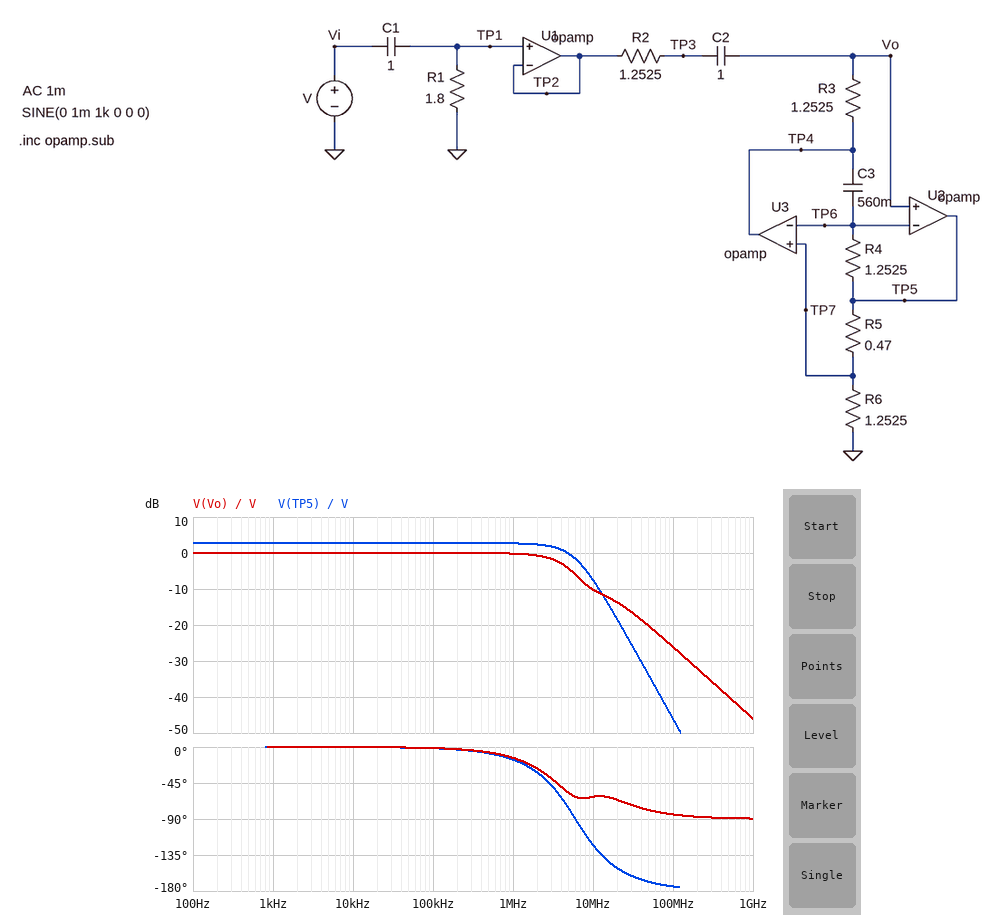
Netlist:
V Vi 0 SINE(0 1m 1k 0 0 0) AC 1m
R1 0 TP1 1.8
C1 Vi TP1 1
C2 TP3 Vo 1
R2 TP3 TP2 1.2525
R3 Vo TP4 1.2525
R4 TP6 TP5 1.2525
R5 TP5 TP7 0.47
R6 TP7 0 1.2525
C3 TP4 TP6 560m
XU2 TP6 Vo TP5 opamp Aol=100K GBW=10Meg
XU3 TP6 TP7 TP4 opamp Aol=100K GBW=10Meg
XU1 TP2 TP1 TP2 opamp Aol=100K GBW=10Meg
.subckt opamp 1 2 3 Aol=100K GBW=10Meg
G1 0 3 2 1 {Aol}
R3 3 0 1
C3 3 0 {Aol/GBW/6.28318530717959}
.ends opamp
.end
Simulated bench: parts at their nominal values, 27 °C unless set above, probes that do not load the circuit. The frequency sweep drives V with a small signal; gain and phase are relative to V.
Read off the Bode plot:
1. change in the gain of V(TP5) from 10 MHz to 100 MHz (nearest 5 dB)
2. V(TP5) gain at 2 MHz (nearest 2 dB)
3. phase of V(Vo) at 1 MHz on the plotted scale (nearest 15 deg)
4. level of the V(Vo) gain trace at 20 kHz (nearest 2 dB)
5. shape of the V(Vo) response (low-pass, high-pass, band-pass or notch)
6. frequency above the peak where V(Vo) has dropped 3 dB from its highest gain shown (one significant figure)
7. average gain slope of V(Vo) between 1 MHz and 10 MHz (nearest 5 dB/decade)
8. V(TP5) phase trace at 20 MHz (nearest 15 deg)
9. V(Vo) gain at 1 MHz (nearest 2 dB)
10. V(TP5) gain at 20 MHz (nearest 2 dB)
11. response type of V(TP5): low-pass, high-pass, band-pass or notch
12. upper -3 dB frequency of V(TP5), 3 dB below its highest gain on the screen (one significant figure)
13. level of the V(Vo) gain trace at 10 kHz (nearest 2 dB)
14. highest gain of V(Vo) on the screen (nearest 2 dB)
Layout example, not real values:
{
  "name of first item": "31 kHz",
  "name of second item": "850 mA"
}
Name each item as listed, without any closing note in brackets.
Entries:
{
  "change in the gain of V(TP5) from 10 MHz to 100 MHz": "-40 dB",
  "V(TP5) gain at 2 MHz": "2 dB",
  "phase of V(Vo) at 1 MHz on the plotted scale": "-15 deg",
  "level of the V(Vo) gain trace at 20 kHz": "0 dB",
  "shape of the V(Vo) response": "low-pass",
  "frequency above the peak where V(Vo) has dropped 3 dB from its highest gain shown": "4 MHz",
  "average gain slope of V(Vo) between 1 MHz and 10 MHz": "-10 dB/decade",
  "V(TP5) phase trace at 20 MHz": "-150 deg",
  "V(Vo) gain at 1 MHz": "0 dB",
  "V(TP5) gain at 20 MHz": "-18 dB",
  "response type of V(TP5): low-pass, high-pass, band-pass or notch": "low-pass",
  "upper -3 dB frequency of V(TP5), 3 dB below its highest gain on the screen": "5 MHz",
  "level of the V(Vo) gain trace at 10 kHz": "0 dB",
  "highest gain of V(Vo) on the screen": "0 dB"
}
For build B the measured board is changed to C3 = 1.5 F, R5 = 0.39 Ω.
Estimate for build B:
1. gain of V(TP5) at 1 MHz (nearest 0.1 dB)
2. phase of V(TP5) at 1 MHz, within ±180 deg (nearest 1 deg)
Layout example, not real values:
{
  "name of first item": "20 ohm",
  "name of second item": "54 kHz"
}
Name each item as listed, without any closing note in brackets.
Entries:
{
  "gain of V(TP5) at 1 MHz": "2.3 dB",
  "phase of V(TP5) at 1 MHz, within ±180 deg": "-15 deg"
}
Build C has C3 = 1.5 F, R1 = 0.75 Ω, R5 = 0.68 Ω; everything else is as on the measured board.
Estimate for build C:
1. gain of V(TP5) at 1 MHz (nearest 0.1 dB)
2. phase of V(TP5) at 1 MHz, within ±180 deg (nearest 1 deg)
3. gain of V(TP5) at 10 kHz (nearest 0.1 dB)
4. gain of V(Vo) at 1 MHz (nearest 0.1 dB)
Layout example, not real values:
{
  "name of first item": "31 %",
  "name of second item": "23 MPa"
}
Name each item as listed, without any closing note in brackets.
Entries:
{
  "gain of V(TP5) at 1 MHz": "3.6 dB",
  "phase of V(TP5) at 1 MHz, within ±180 deg": "-18 deg",
  "gain of V(TP5) at 10 kHz": "3.8 dB",
  "gain of V(Vo) at 1 MHz": "-0.2 dB"
}
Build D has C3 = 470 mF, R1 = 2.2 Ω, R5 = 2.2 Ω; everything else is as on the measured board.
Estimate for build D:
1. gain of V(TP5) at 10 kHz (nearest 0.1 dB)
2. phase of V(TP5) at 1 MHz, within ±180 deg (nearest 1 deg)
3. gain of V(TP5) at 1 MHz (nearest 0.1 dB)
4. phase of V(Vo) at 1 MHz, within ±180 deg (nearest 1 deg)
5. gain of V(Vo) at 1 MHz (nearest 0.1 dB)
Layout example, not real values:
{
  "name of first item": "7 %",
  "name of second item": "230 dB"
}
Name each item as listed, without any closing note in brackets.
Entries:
{
  "gain of V(TP5) at 10 kHz": "8.8 dB",
  "phase of V(TP5) at 1 MHz, within ±180 deg": "-30 deg",
  "gain of V(TP5) at 1 MHz": "8.0 dB",
  "phase of V(Vo) at 1 MHz, within ±180 deg": "-20 deg",
  "gain of V(Vo) at 1 MHz": "-0.7 dB"
}
